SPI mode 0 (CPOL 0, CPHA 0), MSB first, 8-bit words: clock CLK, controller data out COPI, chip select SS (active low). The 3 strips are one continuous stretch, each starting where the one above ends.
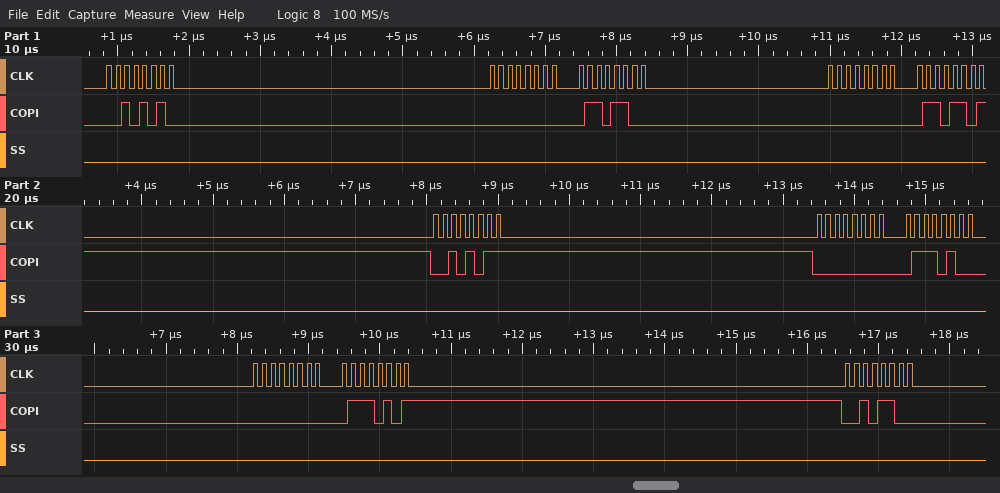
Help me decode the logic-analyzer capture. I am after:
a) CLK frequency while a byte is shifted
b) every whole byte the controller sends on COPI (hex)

8 MHz
2A 00 6C 00 6D 2B 00 74 00 75 2C
